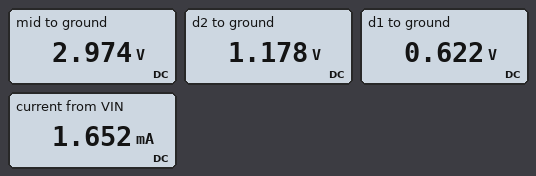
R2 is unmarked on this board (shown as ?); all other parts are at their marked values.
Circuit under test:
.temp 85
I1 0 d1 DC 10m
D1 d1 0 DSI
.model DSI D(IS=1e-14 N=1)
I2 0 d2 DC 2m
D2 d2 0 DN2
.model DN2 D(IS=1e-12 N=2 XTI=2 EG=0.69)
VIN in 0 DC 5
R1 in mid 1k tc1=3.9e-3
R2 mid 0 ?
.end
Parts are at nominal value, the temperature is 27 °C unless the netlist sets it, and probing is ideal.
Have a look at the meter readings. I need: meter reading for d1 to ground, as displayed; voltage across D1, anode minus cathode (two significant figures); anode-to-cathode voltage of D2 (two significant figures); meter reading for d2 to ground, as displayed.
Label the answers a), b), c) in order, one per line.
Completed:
a) 0.622 V
b) 620 mV
c) 1.2 V
d) 1.178 V
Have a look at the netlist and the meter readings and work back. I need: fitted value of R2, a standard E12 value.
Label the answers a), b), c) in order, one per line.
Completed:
a) 1.8 kΩ
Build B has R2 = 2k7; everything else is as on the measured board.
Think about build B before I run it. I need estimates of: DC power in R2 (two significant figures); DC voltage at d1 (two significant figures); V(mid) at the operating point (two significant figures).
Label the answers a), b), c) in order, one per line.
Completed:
a) 4.4 mW
b) 620 mV
c) 3.4 V
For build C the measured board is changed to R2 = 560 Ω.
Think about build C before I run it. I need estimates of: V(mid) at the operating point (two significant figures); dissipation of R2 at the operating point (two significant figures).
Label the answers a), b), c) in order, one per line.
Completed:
a) 1.6 V
b) 4.4 mW
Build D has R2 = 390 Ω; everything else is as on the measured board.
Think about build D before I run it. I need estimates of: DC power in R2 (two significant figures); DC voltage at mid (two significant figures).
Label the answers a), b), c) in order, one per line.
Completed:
a) 3.7 mW
b) 1.2 V
